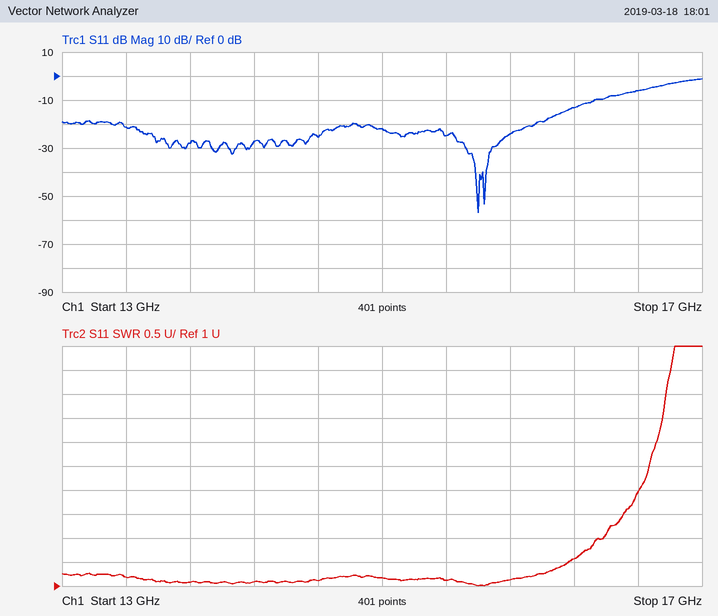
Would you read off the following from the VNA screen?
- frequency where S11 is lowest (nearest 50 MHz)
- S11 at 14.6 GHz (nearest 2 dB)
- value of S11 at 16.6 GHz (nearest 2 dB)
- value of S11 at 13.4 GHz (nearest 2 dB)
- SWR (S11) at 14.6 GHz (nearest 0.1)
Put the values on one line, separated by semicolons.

15.60 GHz; -26 dB; -6 dB; -22 dB; 1.1
